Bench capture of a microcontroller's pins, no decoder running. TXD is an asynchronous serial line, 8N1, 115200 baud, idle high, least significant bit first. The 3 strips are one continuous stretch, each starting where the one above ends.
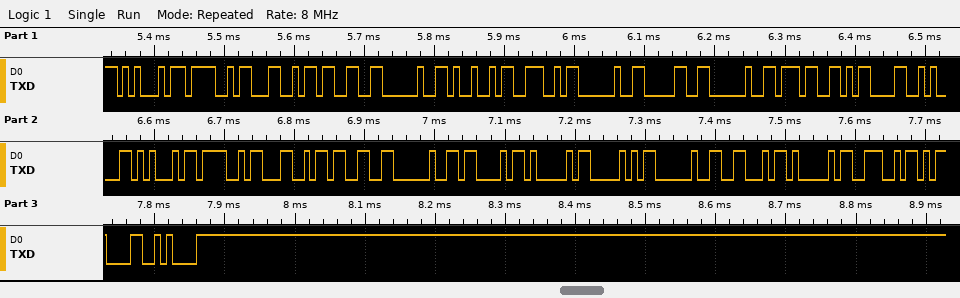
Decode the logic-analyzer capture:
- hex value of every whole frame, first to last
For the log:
45 4F 4C 33 20 49 4E 20 30 20 37 0D 0A 45 4F 4C 33 20 43 41 50 20 46 41 4E 0D 0A
